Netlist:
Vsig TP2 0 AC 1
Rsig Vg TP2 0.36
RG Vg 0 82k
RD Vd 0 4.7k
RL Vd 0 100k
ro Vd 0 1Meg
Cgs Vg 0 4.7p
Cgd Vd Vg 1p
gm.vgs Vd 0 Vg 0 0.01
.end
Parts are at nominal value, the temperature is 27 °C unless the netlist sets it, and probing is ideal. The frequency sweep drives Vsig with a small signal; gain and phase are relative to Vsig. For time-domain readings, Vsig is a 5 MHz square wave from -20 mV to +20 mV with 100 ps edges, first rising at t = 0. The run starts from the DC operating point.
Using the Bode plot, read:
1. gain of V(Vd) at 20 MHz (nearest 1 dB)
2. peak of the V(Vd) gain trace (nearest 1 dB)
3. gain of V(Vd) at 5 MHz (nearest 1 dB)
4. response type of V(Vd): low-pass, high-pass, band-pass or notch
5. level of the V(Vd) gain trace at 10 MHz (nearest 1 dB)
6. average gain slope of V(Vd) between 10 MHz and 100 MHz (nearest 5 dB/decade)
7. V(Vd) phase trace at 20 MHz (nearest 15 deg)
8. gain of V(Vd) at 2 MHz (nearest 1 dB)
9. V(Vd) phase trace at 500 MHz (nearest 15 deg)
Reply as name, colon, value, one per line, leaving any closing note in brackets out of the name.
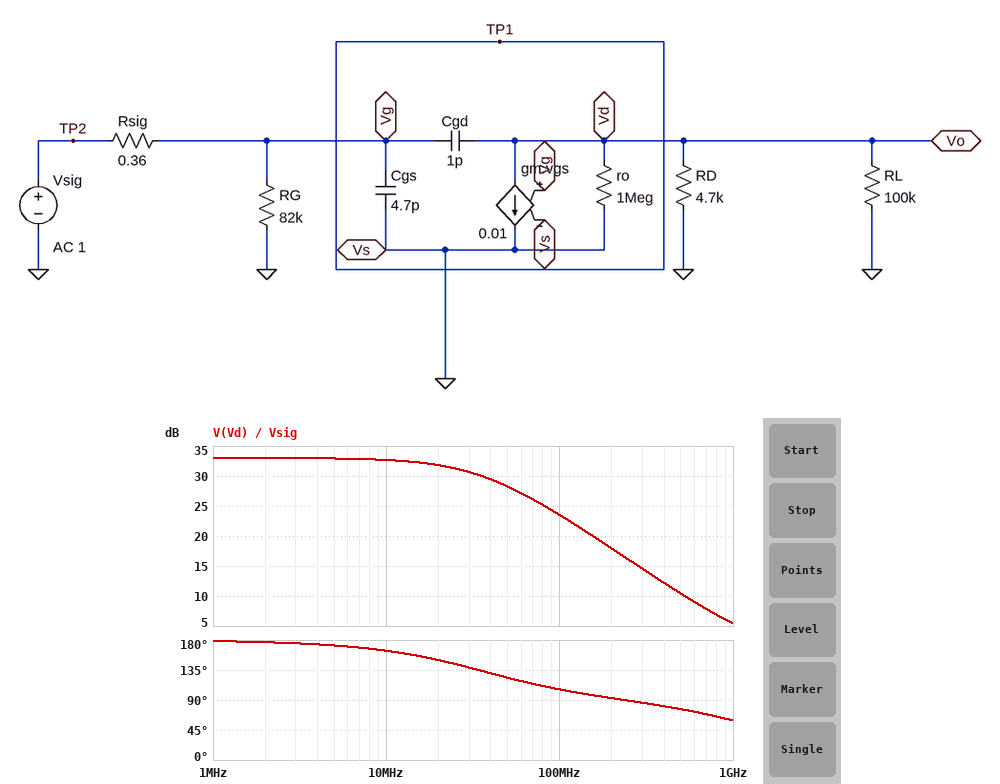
gain of V(Vd) at 20 MHz: 32 dB
peak of the V(Vd) gain trace: 33 dB
gain of V(Vd) at 5 MHz: 33 dB
response type of V(Vd): low-pass, high-pass, band-pass or notch: low-pass
level of the V(Vd) gain trace at 10 MHz: 33 dB
average gain slope of V(Vd) between 10 MHz and 100 MHz: -10 dB/decade
V(Vd) phase trace at 20 MHz: 150 deg
gain of V(Vd) at 2 MHz: 33 dB
V(Vd) phase trace at 500 MHz: 75 deg
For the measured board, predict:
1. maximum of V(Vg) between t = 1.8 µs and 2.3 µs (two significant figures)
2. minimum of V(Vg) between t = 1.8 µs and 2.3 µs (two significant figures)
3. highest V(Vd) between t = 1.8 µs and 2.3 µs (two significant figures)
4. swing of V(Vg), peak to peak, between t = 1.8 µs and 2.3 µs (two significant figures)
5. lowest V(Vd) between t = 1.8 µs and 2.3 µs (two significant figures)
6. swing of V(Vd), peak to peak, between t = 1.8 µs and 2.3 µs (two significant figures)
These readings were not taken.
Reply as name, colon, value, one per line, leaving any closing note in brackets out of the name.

maximum of V(Vg) between t = 1.8 µs and 2.3 µs: 20 mV
minimum of V(Vg) between t = 1.8 µs and 2.3 µs: -20 mV
highest V(Vd) between t = 1.8 µs and 2.3 µs: 910 mV
swing of V(Vg), peak to peak, between t = 1.8 µs and 2.3 µs: 40 mV
lowest V(Vd) between t = 1.8 µs and 2.3 µs: -910 mV
swing of V(Vd), peak to peak, between t = 1.8 µs and 2.3 µs: 1.8 V
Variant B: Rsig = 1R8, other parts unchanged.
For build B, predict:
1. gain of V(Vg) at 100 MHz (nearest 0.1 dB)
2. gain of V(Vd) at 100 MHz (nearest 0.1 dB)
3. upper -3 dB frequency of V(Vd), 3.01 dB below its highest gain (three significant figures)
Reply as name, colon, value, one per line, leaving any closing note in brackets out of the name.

gain of V(Vg) at 100 MHz: -0.1 dB
gain of V(Vd) at 100 MHz: 23.4 dB
upper -3 dB frequency of V(Vd), 3.01 dB below its highest gain: 35.0 MHz
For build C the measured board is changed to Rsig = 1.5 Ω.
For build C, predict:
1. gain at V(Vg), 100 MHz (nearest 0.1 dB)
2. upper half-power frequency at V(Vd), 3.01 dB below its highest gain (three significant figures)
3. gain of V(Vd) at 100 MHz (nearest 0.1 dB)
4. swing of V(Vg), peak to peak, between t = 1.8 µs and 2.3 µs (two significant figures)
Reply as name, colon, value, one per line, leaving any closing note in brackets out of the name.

gain at V(Vg), 100 MHz: -0.1 dB
upper half-power frequency at V(Vd), 3.01 dB below its highest gain: 35.1 MHz
gain of V(Vd) at 100 MHz: 23.4 dB
swing of V(Vg), peak to peak, between t = 1.8 µs and 2.3 µs: 40 mV
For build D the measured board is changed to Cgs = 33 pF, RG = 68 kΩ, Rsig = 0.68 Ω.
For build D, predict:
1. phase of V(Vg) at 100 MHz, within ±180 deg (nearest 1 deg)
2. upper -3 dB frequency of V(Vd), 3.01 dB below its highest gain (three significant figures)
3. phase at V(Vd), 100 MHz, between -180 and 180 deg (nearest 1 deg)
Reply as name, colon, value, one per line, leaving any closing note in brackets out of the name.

phase of V(Vg) at 100 MHz, within ±180 deg: -1 deg
upper -3 dB frequency of V(Vd), 3.01 dB below its highest gain: 35.4 MHz
phase at V(Vd), 100 MHz, between -180 and 180 deg: 105 deg
